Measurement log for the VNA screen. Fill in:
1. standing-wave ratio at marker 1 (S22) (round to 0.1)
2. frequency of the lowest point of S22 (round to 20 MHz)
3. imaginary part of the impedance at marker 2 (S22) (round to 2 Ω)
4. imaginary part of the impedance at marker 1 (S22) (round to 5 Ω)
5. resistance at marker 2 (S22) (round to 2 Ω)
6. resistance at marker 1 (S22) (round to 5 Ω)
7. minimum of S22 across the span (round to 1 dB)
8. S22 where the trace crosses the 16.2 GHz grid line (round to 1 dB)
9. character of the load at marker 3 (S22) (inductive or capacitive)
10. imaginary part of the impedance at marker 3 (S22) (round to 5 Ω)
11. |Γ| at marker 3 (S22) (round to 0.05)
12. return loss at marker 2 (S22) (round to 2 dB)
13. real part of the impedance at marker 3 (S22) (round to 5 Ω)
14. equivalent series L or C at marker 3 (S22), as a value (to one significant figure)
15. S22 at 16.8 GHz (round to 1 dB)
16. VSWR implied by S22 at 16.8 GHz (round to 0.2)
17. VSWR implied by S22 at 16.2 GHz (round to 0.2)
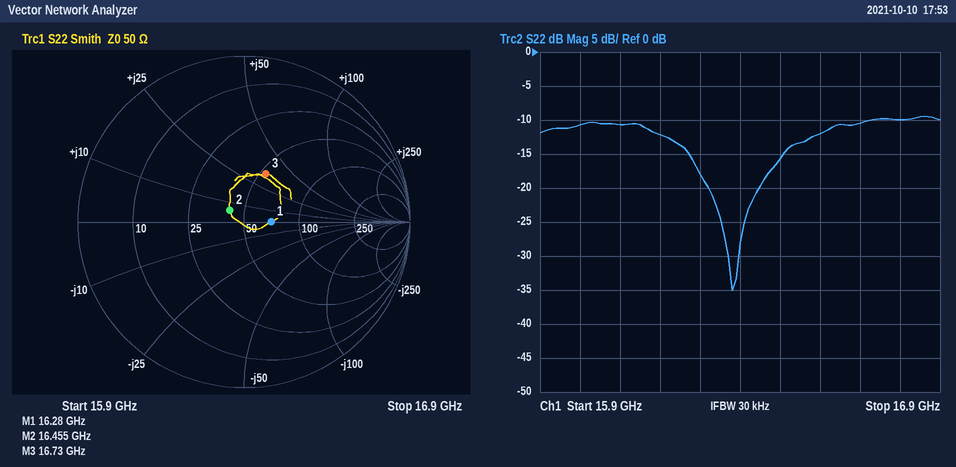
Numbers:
1.4
16.38 GHz
+6 Ω
0 Ω
42 Ω
70 Ω
-35 dB
-12 dB
inductive
+35 Ω
0.30
20 dB
55 Ω
300 pH
-10 dB
2.0
1.6
